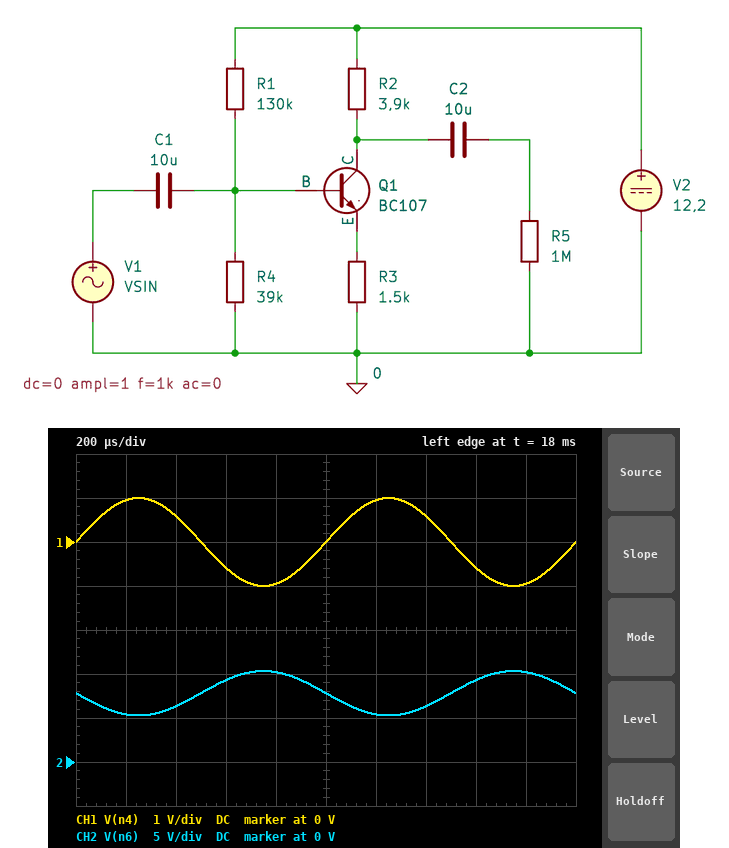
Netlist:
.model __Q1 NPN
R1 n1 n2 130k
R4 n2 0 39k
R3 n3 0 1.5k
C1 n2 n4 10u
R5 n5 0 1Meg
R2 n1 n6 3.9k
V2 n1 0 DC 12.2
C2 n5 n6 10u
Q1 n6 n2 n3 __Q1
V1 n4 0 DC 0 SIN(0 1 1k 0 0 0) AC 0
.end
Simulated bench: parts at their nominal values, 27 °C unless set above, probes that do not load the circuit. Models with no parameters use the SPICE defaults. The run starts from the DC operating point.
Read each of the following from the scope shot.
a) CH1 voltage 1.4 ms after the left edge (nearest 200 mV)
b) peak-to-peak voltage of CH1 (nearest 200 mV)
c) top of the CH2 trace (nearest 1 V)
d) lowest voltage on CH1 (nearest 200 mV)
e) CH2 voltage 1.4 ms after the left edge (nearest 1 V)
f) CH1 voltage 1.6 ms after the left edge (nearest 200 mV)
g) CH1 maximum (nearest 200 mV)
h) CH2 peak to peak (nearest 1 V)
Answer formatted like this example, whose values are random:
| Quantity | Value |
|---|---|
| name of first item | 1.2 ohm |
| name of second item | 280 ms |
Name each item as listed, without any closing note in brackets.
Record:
| Quantity | Value |
|---|---|
| CH1 voltage 1.4 ms after the left edge | 600 mV |
| peak-to-peak voltage of CH1 | 2.0 V |
| top of the CH2 trace | 10 V |
| lowest voltage on CH1 | -1.0 V |
| CH2 voltage 1.4 ms after the left edge | 6 V |
| CH1 voltage 1.6 ms after the left edge | -600 mV |
| CH1 maximum | 1.0 V |
| CH2 peak to peak | 5 V |
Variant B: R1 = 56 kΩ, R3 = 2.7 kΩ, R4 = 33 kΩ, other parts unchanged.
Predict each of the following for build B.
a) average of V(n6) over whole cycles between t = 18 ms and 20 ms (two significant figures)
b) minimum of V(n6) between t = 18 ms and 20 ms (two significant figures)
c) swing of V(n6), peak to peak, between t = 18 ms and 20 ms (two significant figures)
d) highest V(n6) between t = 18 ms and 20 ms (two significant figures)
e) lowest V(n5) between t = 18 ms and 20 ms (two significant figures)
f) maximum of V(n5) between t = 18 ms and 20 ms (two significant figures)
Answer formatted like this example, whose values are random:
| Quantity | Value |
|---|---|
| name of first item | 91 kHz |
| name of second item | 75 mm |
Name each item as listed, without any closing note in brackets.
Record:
| Quantity | Value |
|---|---|
| average of V(n6) over whole cycles between t = 18 ms and 20 ms | 7.2 V |
| minimum of V(n6) between t = 18 ms and 20 ms | 5.8 V |
| swing of V(n6), peak to peak, between t = 18 ms and 20 ms | 2.8 V |
| highest V(n6) between t = 18 ms and 20 ms | 8.6 V |
| lowest V(n5) between t = 18 ms and 20 ms | -1.4 V |
| maximum of V(n5) between t = 18 ms and 20 ms | 1.4 V |
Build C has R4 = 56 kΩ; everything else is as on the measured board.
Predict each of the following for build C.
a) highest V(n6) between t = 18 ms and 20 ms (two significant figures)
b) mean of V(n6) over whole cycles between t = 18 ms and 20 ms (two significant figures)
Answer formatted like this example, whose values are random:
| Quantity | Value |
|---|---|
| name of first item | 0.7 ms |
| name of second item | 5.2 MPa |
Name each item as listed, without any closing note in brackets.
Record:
| Quantity | Value |
|---|---|
| highest V(n6) between t = 18 ms and 20 ms | 8.8 V |
| mean of V(n6) over whole cycles between t = 18 ms and 20 ms | 6.3 V |
